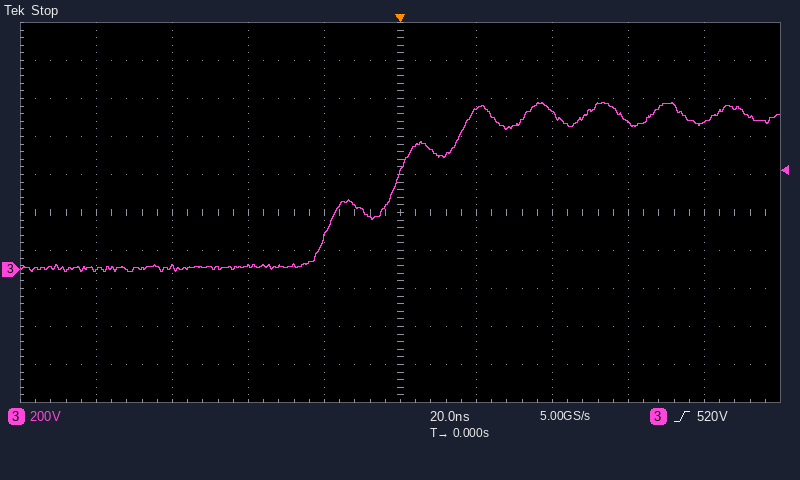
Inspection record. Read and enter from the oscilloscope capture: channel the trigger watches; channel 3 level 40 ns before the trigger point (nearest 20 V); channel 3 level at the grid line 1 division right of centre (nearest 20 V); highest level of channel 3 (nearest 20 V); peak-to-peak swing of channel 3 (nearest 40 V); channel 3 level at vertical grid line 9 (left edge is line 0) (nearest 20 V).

channel 3
20 V
840 V
880 V
880 V
780 V
